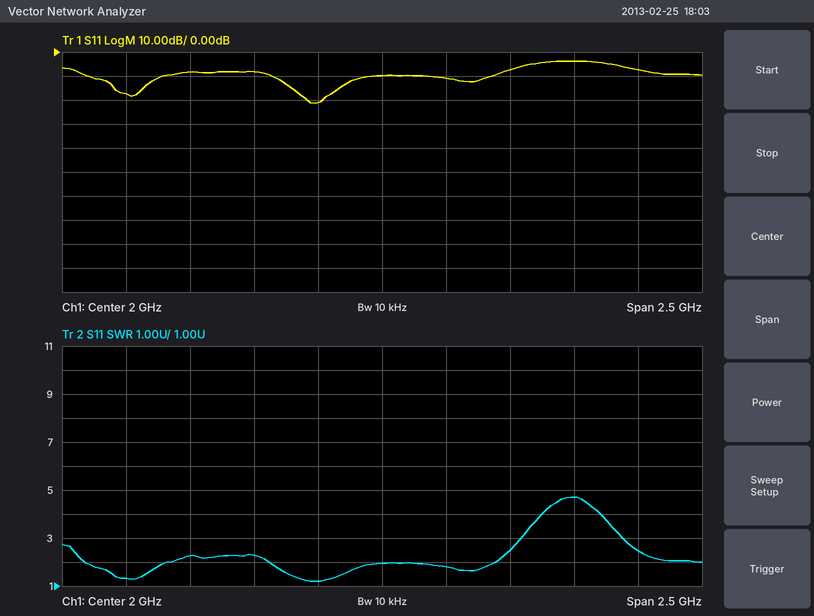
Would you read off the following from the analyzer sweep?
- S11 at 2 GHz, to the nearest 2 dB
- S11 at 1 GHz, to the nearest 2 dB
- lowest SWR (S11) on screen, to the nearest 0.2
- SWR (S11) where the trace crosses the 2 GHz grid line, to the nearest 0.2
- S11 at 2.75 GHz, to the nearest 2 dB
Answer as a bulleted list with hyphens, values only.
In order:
- -10 dB
- -18 dB
- 1.2
- 2.0
- -4 dB
